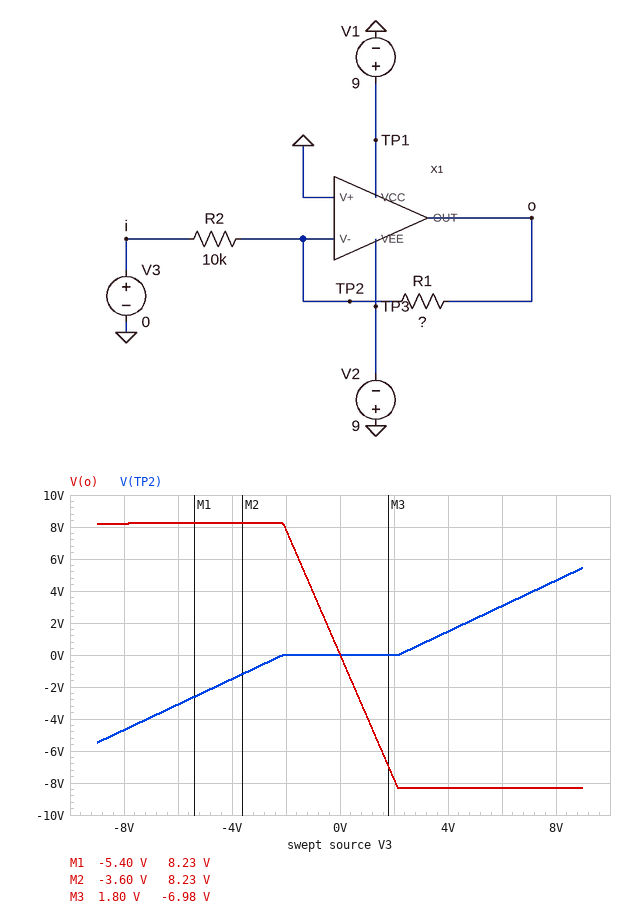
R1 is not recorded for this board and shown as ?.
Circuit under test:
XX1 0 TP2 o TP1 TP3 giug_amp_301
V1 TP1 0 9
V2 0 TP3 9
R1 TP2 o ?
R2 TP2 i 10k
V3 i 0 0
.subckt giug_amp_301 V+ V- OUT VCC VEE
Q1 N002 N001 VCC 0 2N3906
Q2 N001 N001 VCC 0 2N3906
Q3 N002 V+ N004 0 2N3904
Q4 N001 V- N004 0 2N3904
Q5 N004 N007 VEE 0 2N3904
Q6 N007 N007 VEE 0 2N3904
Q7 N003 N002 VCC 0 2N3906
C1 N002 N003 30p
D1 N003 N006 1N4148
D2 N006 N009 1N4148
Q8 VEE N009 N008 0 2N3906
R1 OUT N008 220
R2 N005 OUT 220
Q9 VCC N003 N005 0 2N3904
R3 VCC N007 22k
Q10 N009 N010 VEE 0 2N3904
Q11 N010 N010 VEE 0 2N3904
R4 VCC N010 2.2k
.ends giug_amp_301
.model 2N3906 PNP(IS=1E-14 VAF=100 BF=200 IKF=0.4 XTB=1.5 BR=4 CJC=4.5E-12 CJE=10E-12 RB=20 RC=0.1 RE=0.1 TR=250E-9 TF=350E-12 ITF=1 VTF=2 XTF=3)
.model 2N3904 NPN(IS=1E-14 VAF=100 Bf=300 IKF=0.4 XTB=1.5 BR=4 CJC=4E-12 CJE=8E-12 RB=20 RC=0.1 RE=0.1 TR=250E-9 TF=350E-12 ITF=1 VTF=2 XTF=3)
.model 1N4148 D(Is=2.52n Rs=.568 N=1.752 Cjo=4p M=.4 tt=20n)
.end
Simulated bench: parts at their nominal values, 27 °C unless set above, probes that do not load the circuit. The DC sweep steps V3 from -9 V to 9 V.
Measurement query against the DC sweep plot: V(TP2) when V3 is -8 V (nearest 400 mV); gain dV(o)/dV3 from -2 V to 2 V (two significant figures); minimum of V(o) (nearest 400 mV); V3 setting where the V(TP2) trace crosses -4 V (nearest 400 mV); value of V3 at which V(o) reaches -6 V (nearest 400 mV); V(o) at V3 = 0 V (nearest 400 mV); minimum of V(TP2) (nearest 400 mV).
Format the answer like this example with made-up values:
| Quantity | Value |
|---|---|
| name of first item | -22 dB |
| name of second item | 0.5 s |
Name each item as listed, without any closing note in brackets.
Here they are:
| Quantity | Value |
|---|---|
| V(TP2) when V3 is -8 V | -4.8 V |
| gain dV(o)/dV3 from -2 V to 2 V | -3.9 V/V |
| minimum of V(o) | -8.4 V |
| V3 setting where the V(TP2) trace crosses -4 V | -7.2 V |
| value of V3 at which V(o) reaches -6 V | 1.6 V |
| V(o) at V3 = 0 V | 0 V |
| minimum of V(TP2) | -5.6 V |
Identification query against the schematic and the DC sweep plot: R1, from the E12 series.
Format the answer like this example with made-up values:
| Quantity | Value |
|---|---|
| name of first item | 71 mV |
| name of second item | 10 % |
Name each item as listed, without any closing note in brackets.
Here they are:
| Quantity | Value |
|---|---|
| R1, from the E12 series | 39 kΩ |
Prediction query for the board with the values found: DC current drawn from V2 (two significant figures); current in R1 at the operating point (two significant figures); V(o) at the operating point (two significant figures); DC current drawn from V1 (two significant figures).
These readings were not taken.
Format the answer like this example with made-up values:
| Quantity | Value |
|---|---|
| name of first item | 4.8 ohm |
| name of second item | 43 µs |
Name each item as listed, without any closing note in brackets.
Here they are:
| Quantity | Value |
|---|---|
| DC current drawn from V2 | 18 mA |
| current in R1 at the operating point | 1.0 µA |
| V(o) at the operating point | 37 mV |
| DC current drawn from V1 | 18 mA |
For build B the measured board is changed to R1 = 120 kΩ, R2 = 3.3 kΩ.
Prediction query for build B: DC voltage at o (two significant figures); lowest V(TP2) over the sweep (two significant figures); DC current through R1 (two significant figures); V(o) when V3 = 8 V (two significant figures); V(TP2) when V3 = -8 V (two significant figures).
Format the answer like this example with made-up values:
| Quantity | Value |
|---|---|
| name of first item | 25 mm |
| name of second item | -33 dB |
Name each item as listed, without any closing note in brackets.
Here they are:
| Quantity | Value |
|---|---|
| DC voltage at o | 65 mV |
| lowest V(TP2) over the sweep | -8.5 V |
| DC current through R1 | 560 nA |
| V(o) when V3 = 8 V | -8.4 V |
| V(TP2) when V3 = -8 V | -7.6 V |
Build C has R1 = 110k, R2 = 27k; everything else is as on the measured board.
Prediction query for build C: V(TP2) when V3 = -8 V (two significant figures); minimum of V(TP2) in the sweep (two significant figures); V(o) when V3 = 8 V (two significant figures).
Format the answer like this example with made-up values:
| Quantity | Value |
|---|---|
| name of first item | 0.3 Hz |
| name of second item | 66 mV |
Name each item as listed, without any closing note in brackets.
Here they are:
| Quantity | Value |
|---|---|
| V(TP2) when V3 = -8 V | -4.8 V |
| minimum of V(TP2) in the sweep | -5.6 V |
| V(o) when V3 = 8 V | -8.4 V |
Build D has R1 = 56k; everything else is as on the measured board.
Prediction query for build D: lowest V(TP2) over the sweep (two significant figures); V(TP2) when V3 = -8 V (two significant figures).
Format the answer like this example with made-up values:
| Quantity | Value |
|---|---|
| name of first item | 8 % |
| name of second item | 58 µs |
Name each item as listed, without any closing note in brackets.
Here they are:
| Quantity | Value |
|---|---|
| lowest V(TP2) over the sweep | -6.4 V |
| V(TP2) when V3 = -8 V | -5.5 V |
